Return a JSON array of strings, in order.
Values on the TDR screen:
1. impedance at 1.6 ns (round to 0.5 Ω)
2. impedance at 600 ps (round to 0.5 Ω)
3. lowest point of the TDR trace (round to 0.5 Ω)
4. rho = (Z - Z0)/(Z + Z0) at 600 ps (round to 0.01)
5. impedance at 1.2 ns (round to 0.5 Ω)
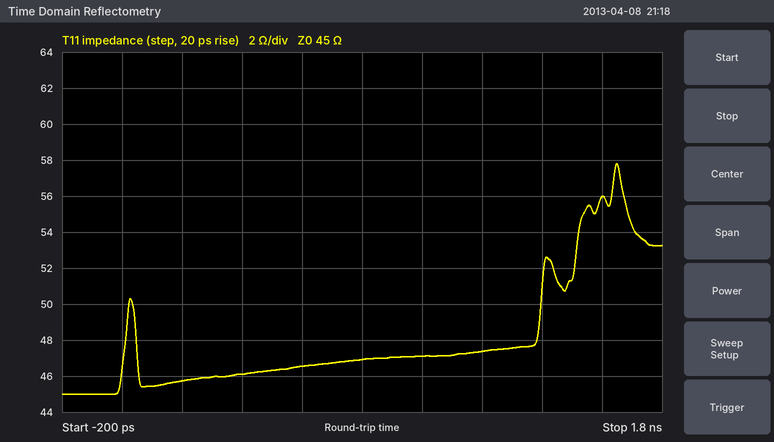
["56.0 Ω", "46.5 Ω", "45.0 Ω", "+0.02", "47.5 Ω"]
